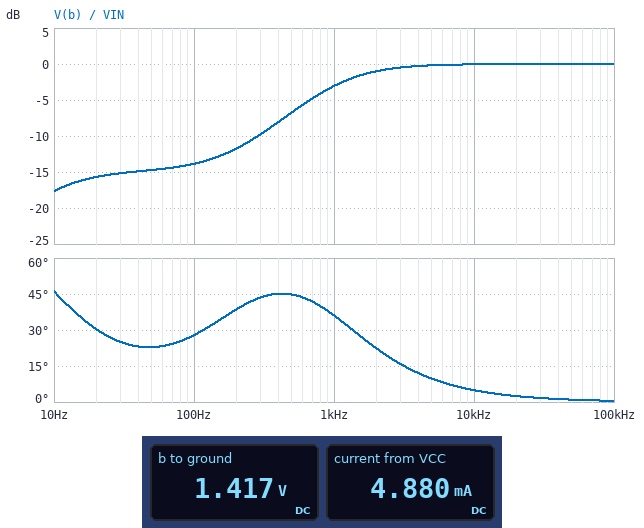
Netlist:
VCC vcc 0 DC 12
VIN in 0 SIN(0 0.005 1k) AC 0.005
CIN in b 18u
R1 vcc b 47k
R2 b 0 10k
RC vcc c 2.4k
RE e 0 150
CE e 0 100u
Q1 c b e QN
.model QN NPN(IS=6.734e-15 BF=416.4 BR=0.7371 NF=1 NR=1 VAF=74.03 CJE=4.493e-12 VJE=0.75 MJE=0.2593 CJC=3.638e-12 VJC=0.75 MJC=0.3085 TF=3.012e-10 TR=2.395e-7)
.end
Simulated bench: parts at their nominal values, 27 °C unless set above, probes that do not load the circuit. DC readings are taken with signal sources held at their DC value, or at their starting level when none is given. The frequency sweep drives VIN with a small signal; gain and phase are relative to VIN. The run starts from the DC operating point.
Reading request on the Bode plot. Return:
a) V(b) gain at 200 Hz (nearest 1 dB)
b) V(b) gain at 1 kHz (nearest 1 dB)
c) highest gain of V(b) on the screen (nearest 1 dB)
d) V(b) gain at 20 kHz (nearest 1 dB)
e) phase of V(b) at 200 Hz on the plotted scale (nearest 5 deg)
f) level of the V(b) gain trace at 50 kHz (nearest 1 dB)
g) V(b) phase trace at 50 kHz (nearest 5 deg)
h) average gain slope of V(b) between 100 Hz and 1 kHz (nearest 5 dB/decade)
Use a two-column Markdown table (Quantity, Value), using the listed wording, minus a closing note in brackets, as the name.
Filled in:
| Quantity | Value |
|---|---|
| V(b) gain at 200 Hz | -12 dB |
| V(b) gain at 1 kHz | -3 dB |
| highest gain of V(b) on the screen | 0 dB |
| V(b) gain at 20 kHz | 0 dB |
| phase of V(b) at 200 Hz on the plotted scale | 40 deg |
| level of the V(b) gain trace at 50 kHz | 0 dB |
| V(b) phase trace at 50 kHz | 0 deg |
| average gain slope of V(b) between 100 Hz and 1 kHz | 10 dB/decade |
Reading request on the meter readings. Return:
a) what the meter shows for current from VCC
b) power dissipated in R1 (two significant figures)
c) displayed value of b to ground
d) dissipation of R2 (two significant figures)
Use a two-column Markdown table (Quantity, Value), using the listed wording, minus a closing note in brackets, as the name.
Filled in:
| Quantity | Value |
|---|---|
| what the meter shows for current from VCC | 4.880 mA |
| power dissipated in R1 | 2.4 mW |
| displayed value of b to ground | 1.417 V |
| dissipation of R2 | 200 µW |
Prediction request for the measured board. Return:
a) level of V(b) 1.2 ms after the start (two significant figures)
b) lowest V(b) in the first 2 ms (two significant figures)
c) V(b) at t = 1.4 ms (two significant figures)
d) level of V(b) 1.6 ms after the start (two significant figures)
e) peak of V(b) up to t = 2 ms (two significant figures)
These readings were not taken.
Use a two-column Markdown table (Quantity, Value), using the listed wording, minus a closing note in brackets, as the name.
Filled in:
| Quantity | Value |
|---|---|
| level of V(b) 1.2 ms after the start | 1.4 V |
| lowest V(b) in the first 2 ms | 1.4 V |
| V(b) at t = 1.4 ms | 1.4 V |
| level of V(b) 1.6 ms after the start | 1.4 V |
| peak of V(b) up to t = 2 ms | 1.4 V |
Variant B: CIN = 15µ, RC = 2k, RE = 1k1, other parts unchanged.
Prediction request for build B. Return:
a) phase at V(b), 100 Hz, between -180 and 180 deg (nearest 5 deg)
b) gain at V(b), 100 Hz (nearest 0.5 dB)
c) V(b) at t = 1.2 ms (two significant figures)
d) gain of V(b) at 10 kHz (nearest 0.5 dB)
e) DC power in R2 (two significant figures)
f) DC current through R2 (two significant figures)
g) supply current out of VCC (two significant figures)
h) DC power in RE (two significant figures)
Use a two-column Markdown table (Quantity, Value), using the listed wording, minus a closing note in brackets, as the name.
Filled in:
| Quantity | Value |
|---|---|
| phase at V(b), 100 Hz, between -180 and 180 deg | 0 deg |
| gain at V(b), 100 Hz | 0 dB |
| V(b) at t = 1.2 ms | 2.1 V |
| gain of V(b) at 10 kHz | 0 dB |
| DC power in R2 | 430 µW |
| DC current through R2 | 210 µA |
| supply current out of VCC | 1.5 mA |
| DC power in RE | 1.8 mW |
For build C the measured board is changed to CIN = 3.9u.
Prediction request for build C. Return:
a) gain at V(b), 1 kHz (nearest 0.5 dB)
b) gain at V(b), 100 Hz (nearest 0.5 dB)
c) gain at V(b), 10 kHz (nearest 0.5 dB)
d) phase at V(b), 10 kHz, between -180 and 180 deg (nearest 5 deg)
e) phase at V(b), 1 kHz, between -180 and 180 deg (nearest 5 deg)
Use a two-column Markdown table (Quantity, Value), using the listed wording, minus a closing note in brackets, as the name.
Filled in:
| Quantity | Value |
|---|---|
| gain at V(b), 1 kHz | -12.5 dB |
| gain at V(b), 100 Hz | -26.0 dB |
| gain at V(b), 10 kHz | -0.5 dB |
| phase at V(b), 10 kHz, between -180 and 180 deg | 20 deg |
| phase at V(b), 1 kHz, between -180 and 180 deg | 65 deg |
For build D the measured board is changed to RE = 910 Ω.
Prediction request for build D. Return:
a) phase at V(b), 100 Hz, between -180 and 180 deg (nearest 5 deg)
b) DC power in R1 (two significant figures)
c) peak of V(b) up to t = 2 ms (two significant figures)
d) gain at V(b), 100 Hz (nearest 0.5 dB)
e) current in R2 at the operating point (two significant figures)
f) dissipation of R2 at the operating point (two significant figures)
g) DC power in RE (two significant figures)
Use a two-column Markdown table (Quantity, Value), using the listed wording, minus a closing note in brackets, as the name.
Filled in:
| Quantity | Value |
|---|---|
| phase at V(b), 100 Hz, between -180 and 180 deg | 0 deg |
| DC power in R1 | 2.1 mW |
| peak of V(b) up to t = 2 ms | 2.1 V |
| gain at V(b), 100 Hz | 0 dB |
| current in R2 at the operating point | 210 µA |
| dissipation of R2 at the operating point | 430 µW |
| DC power in RE | 2.2 mW |
